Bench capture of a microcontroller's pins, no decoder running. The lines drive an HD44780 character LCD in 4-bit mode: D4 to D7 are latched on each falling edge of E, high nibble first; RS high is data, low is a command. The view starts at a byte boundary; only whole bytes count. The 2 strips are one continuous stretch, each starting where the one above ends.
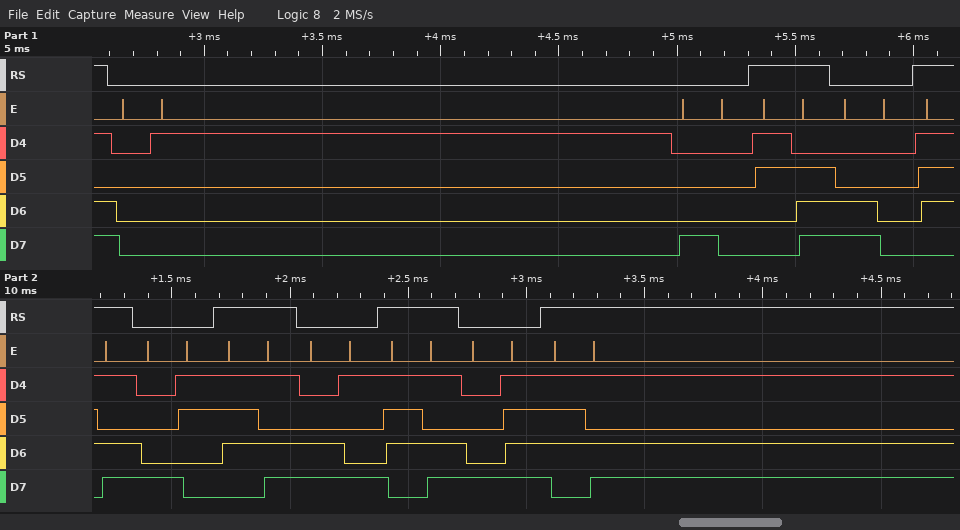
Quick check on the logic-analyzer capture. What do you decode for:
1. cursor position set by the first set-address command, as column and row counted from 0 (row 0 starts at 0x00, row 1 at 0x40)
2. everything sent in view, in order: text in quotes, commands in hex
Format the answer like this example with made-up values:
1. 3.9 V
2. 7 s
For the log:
1. column 0, row 0
2. 0x01 0x80 ">" 0xC0 "}" 0x83 "}" 0xC9 "}" 0x8F "}"
